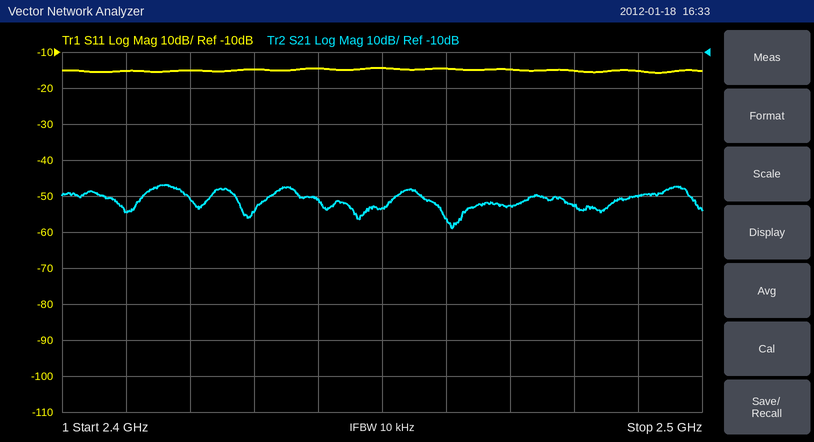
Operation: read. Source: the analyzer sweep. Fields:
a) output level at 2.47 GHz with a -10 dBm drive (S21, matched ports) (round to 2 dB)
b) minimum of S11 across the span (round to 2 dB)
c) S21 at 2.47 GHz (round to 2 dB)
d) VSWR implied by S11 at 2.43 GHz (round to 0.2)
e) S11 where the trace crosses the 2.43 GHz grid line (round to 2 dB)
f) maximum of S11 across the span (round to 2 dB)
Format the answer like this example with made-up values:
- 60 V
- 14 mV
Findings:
- -62 dBm
- -16 dB
- -52 dB
- 1.4
- -14 dB
- -14 dB
